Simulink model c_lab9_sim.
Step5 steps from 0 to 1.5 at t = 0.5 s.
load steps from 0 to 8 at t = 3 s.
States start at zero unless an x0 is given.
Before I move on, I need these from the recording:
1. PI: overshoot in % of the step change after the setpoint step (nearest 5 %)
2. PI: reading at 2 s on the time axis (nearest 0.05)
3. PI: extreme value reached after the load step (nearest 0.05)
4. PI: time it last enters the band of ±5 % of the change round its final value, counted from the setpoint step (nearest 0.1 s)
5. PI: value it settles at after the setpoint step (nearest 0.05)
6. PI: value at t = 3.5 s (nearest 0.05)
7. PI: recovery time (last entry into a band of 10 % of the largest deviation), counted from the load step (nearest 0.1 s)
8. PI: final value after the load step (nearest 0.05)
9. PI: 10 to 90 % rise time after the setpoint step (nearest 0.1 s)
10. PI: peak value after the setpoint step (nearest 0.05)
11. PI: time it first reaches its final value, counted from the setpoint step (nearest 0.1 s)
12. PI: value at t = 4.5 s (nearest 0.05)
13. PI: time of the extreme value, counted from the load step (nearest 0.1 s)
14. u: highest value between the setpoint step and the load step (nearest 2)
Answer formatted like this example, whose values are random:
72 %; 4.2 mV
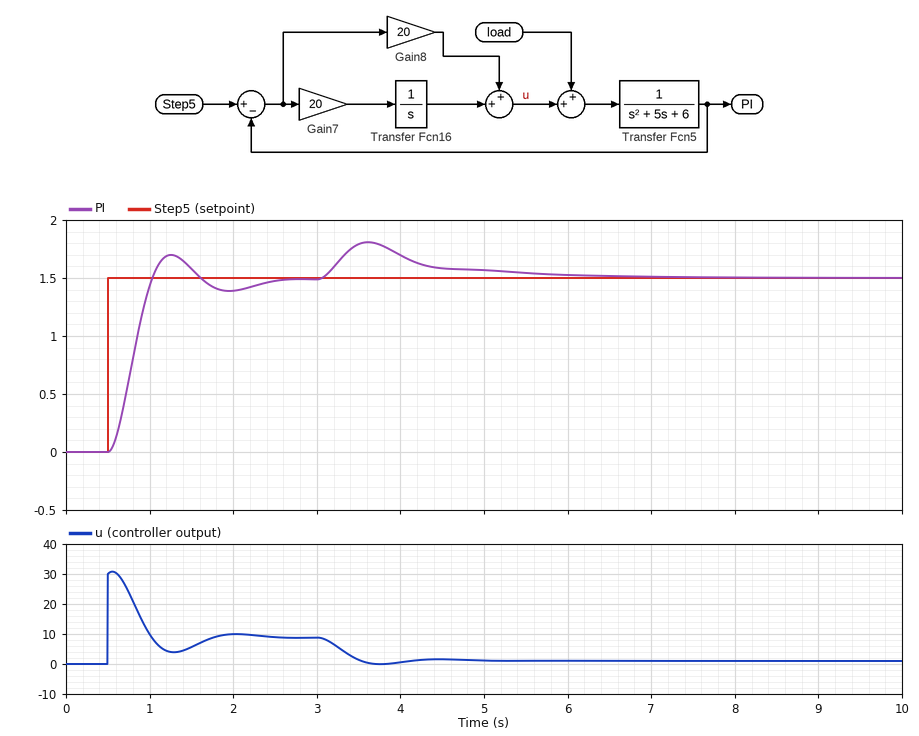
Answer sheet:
15 %; 1.40; 1.80; 1.7 s; 1.50; 1.80; 2.8 s; 1.50; 0.4 s; 1.70; 0.5 s; 1.60; 0.6 s; 30
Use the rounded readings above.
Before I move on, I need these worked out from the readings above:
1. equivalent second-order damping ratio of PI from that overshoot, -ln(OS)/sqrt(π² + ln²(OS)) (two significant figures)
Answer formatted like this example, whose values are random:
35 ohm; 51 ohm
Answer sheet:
0.52
